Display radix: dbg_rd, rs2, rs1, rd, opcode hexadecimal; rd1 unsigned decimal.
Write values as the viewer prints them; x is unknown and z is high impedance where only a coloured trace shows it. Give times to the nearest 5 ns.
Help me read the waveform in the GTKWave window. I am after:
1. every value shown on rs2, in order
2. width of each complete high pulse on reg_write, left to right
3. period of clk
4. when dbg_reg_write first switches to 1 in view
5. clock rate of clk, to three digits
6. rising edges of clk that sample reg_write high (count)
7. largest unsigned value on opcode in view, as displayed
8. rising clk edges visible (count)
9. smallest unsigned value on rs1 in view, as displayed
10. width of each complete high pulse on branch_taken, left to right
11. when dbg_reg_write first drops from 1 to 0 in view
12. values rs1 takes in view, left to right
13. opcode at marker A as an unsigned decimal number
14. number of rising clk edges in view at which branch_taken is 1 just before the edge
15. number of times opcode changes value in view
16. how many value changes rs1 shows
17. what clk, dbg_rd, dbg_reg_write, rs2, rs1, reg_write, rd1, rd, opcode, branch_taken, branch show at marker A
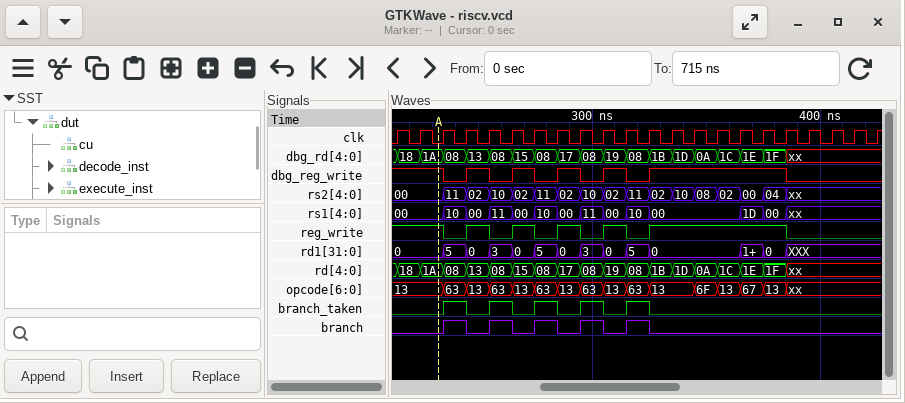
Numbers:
00, 11, 02, 10, 02, 11, 02, 10, 02, 11, 02, 10, 08, 02, 00, 04, xx
10 ns, 10 ns, 10 ns, 10 ns, 60 ns
10 ns
245 ns
100 MHz
13
6F
22
00
10 ns, 10 ns, 10 ns, 10 ns, 10 ns
235 ns
00, 10, 00, 11, 00, 10, 00, 11, 00, 10, 00, 1D, 00, xx
19
5
15
13
clk=0, dbg_rd=1A, dbg_reg_write=1, rs2=00, rs1=00, reg_write=1, rd1=0, rd=1A, opcode=13, branch_taken=0, branch=0
